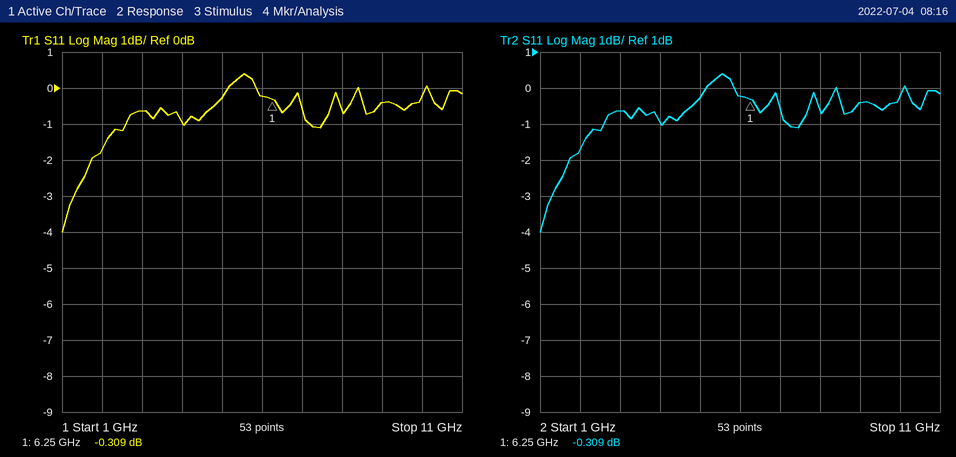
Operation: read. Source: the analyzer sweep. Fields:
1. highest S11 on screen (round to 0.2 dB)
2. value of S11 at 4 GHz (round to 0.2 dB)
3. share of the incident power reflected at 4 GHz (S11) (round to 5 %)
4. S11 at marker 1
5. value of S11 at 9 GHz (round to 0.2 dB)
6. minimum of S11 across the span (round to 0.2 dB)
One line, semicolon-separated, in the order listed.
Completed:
0.4 dB; -1.0 dB; 80 %; -0.309 dB; -0.4 dB; -4.0 dB
